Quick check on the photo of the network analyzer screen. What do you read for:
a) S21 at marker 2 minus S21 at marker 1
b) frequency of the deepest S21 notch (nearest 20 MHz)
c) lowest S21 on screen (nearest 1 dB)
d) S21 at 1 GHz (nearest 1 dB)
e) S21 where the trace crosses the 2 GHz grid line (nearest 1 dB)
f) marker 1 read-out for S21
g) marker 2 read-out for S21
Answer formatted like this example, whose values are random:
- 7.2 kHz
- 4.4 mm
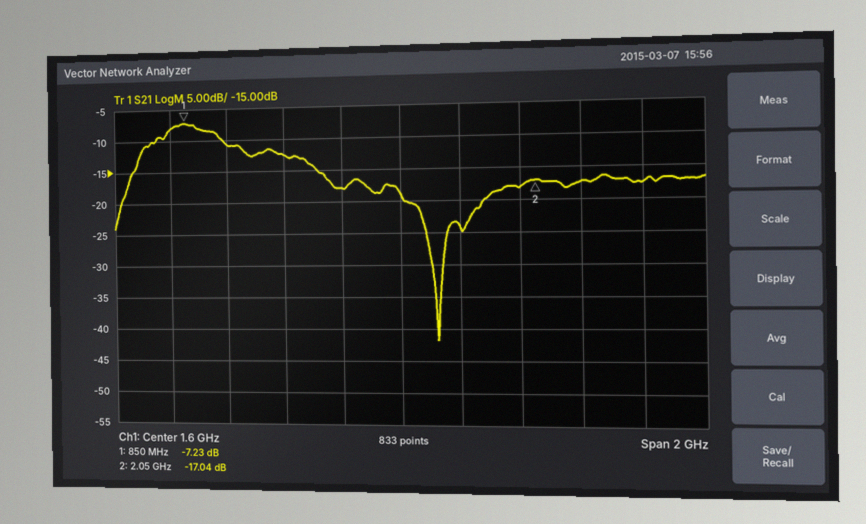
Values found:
- -9.81 dB
- 1.72 GHz
- -42 dB
- -11 dB
- -18 dB
- -7.23 dB
- -17.04 dB
